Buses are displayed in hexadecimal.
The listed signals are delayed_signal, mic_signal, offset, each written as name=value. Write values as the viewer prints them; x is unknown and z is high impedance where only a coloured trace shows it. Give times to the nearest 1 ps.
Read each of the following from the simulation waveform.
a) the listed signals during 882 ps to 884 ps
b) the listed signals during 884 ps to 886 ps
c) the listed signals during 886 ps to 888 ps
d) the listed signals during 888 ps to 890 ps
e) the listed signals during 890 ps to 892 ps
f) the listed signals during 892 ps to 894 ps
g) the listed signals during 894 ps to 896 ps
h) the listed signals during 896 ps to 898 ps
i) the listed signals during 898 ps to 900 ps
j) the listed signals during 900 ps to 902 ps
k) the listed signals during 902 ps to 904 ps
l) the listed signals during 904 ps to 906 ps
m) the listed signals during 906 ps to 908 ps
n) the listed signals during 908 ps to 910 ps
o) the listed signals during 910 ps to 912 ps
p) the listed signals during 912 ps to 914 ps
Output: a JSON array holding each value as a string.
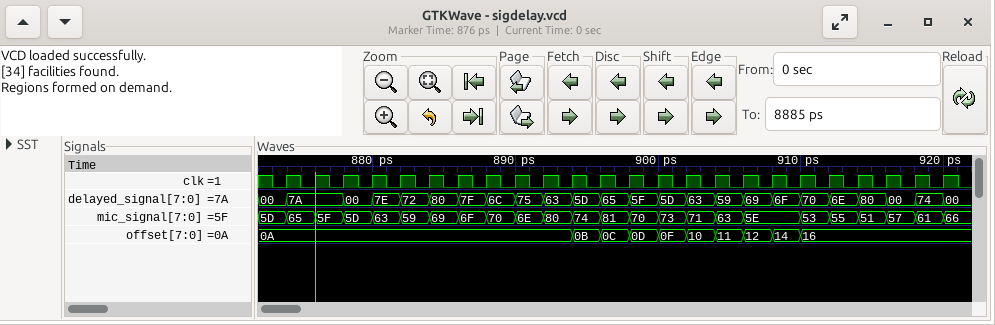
["delayed_signal=72, mic_signal=59, offset=0A", "delayed_signal=80, mic_signal=69, offset=0A", "delayed_signal=7F, mic_signal=6F, offset=0A", "delayed_signal=6C, mic_signal=70, offset=0A", "delayed_signal=75, mic_signal=6E, offset=0A", "delayed_signal=63, mic_signal=80, offset=0A", "delayed_signal=5D, mic_signal=74, offset=0B", "delayed_signal=65, mic_signal=81, offset=0C", "delayed_signal=5F, mic_signal=70, offset=0D", "delayed_signal=5D, mic_signal=73, offset=0F", "delayed_signal=63, mic_signal=71, offset=10", "delayed_signal=59, mic_signal=63, offset=11", "delayed_signal=69, mic_signal=5E, offset=12", "delayed_signal=6F, mic_signal=5E, offset=14", "delayed_signal=70, mic_signal=53, offset=16", "delayed_signal=6E, mic_signal=55, offset=16"]
